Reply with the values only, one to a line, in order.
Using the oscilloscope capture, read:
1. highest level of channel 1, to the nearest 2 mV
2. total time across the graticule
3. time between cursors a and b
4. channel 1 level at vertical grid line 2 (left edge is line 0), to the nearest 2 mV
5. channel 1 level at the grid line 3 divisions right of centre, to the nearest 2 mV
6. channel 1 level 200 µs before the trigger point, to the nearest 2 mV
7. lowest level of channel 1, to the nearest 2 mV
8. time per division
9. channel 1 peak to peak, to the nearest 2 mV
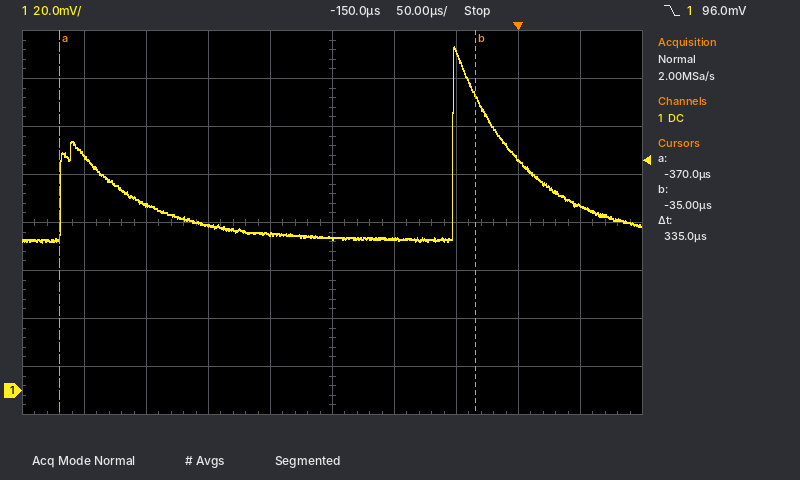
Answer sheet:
144 mV
500 µs
335 µs
78 mV
96 mV
66 mV
62 mV
50 µs
82 mV
